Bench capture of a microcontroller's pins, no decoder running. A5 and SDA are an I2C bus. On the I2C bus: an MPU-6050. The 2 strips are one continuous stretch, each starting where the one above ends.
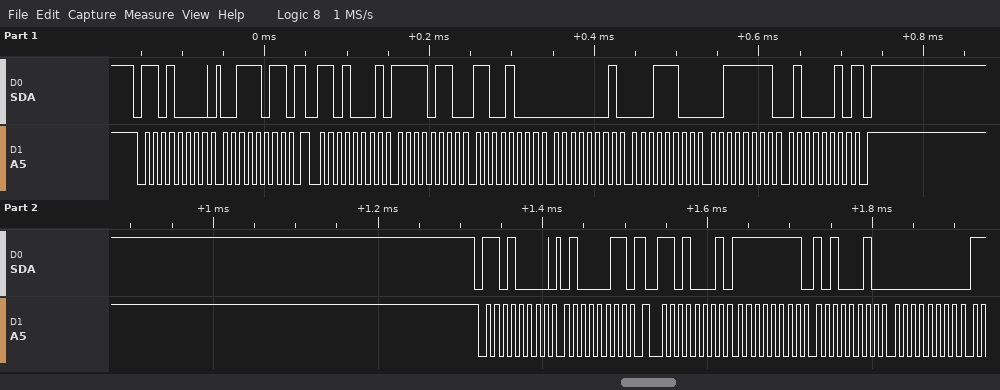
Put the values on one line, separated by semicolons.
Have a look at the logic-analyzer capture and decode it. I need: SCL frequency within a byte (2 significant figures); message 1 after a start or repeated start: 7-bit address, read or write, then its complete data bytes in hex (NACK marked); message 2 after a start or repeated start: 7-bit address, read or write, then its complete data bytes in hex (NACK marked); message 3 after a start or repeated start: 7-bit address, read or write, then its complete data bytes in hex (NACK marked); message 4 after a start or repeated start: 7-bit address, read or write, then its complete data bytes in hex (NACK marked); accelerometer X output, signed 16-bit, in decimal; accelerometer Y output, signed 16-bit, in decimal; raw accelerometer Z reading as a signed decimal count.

100 kHz; 0x68 write: 3B; 0x68 read: F6 C8 01 1C 3F 42 NACK; 0x68 write: 43; 0x68 read: FF A2 00; -2360; 284; 16194
